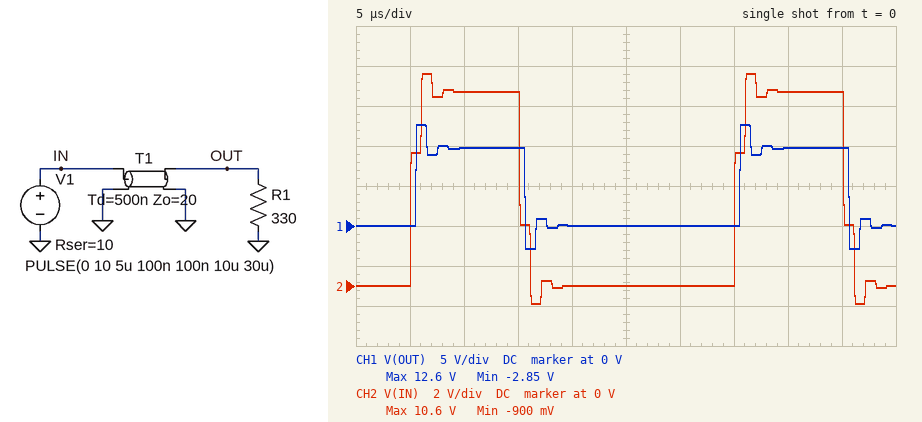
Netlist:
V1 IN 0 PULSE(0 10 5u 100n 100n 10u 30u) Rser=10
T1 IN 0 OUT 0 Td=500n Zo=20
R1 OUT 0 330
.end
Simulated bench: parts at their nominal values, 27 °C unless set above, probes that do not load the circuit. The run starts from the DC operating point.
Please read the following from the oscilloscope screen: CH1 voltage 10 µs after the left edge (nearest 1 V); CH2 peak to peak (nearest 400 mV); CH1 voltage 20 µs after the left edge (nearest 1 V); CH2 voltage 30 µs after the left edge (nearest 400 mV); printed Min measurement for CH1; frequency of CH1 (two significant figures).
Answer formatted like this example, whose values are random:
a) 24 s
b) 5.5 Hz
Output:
a) 10 V
b) 11.6 V
c) 0 V
d) 0 V
e) -2.85 V
f) 33 kHz
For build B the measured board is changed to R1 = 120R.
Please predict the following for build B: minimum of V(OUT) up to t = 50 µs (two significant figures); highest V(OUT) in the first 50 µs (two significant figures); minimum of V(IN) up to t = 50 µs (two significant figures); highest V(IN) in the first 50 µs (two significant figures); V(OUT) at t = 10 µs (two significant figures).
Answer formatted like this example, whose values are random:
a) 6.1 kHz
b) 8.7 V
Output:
a) -2.2 V
b) 11 V
c) -610 mV
d) 9.8 V
e) 9.2 V
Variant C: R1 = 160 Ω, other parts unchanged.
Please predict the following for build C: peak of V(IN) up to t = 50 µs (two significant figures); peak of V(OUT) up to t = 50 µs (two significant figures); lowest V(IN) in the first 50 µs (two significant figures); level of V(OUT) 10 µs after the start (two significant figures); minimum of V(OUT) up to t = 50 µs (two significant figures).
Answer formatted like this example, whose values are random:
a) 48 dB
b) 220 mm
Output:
a) 10 V
b) 12 V
c) -710 mV
d) 9.4 V
e) -2.4 V
